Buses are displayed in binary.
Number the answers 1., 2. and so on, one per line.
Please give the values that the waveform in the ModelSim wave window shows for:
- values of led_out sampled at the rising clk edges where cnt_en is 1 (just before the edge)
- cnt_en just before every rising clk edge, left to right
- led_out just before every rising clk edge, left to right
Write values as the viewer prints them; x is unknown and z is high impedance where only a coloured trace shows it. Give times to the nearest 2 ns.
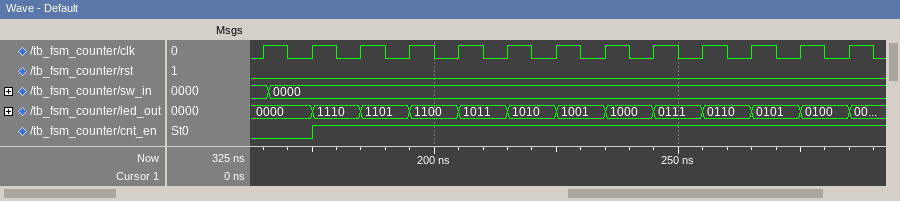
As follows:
1. 1110, 1101, 1100, 1011, 1010, 1001, 1000, 0111, 0110, 0101, 0100
2. 0 0 1 1 1 1 1 1 1 1 1 1 1
3. 0000, 0000, 1110, 1101, 1100, 1011, 1010, 1001, 1000, 0111, 0110, 0101, 0100
